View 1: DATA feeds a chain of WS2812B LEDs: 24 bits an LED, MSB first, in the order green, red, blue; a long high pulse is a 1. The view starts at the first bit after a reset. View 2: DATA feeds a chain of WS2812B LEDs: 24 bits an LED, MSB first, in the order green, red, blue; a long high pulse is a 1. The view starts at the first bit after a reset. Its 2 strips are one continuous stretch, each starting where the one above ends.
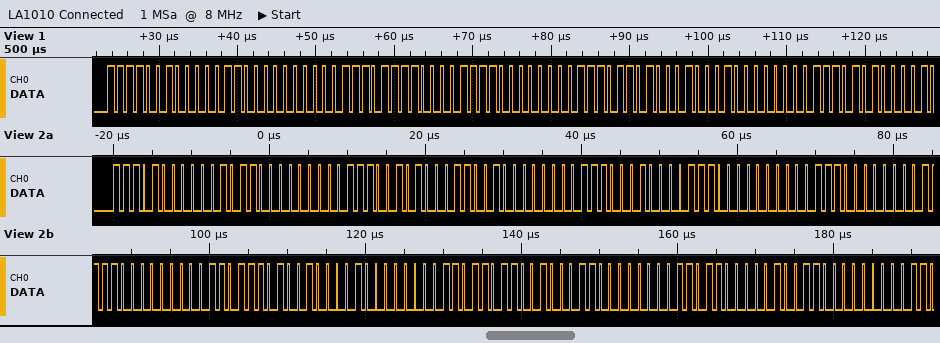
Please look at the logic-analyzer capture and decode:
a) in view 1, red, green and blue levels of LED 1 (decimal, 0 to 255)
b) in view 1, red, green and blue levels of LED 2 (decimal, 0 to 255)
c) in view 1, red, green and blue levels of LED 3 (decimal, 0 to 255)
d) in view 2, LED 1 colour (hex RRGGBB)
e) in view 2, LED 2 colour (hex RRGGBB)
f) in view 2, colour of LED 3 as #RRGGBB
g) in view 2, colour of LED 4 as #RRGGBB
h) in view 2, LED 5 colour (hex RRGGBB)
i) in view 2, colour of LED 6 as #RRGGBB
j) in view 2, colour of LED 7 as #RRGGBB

12, 242, 0
15, 239, 0
17, 237, 0
#16E800
#19E500
#1CE200
#1EE000
#21DD00
#23DB00
#26D800
